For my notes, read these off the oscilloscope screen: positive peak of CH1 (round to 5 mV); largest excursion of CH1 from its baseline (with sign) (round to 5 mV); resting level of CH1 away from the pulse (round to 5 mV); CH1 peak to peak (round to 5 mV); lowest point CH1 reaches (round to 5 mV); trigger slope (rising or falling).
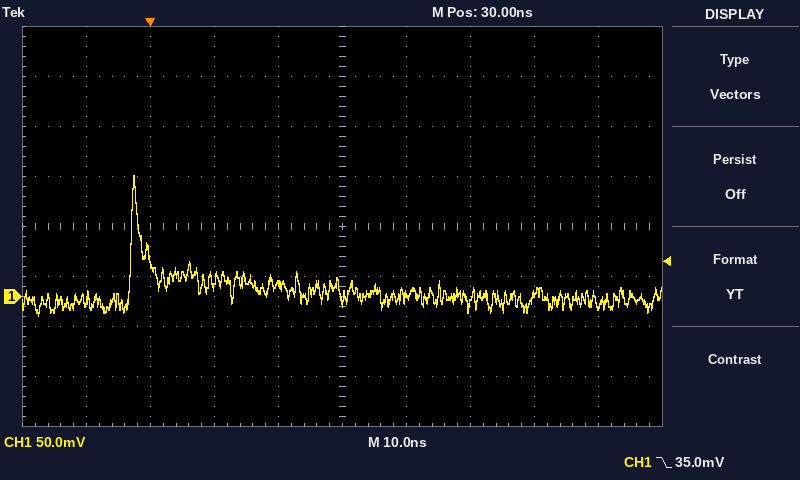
120 mV
+120 mV
0 mV
140 mV
-20 mV
falling
